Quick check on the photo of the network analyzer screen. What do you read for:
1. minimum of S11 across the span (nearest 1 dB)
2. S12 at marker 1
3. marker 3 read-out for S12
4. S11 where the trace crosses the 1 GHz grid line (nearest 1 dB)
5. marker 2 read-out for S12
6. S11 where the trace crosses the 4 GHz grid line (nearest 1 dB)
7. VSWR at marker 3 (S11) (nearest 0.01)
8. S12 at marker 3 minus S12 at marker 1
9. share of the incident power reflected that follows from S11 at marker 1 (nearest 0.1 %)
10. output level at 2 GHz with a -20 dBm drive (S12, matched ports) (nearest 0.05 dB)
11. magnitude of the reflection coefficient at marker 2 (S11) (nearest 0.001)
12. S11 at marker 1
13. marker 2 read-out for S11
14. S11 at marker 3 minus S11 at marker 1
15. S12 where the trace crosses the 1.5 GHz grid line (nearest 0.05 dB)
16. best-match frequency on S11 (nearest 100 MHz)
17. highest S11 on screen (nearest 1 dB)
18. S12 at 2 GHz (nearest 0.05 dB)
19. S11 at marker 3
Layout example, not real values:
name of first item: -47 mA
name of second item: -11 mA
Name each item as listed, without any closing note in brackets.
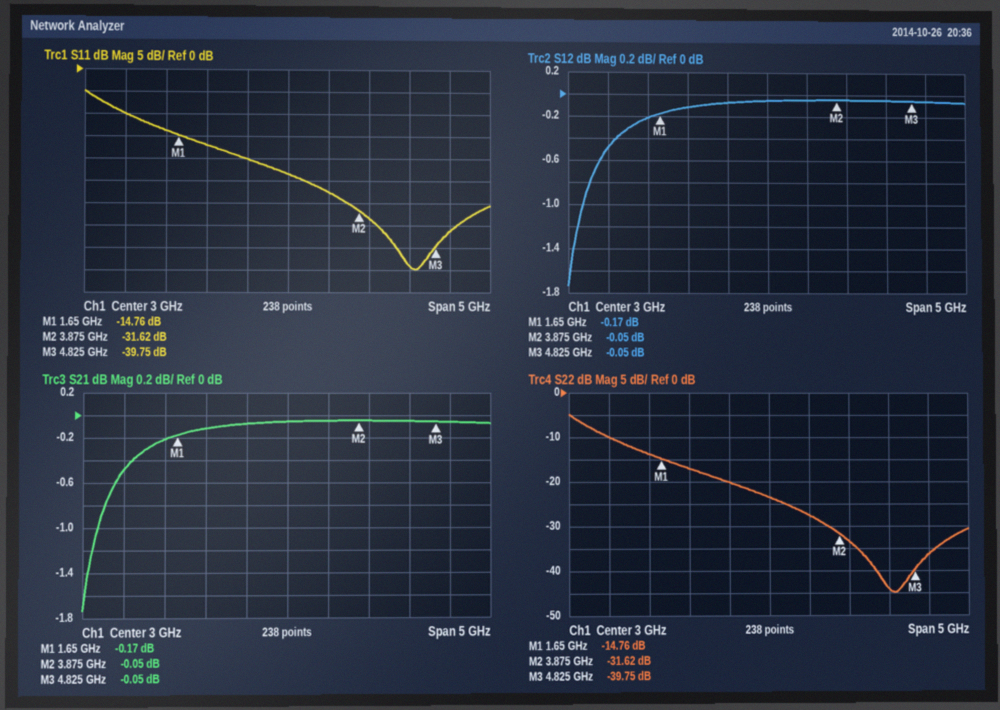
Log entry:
minimum of S11 across the span: -45 dB
S12 at marker 1: -0.17 dB
marker 3 read-out for S12: -0.05 dB
S11 where the trace crosses the 1 GHz grid line: -10 dB
marker 2 read-out for S12: -0.05 dB
S11 where the trace crosses the 4 GHz grid line: -33 dB
VSWR at marker 3 (S11): 1.02
S12 at marker 3 minus S12 at marker 1: 0.12 dB
share of the incident power reflected that follows from S11 at marker 1: 3.3 %
output level at 2 GHz with a -20 dBm drive (S12, matched ports): -20.10 dBm
magnitude of the reflection coefficient at marker 2 (S11): 0.026
S11 at marker 1: -14.76 dB
marker 2 read-out for S11: -31.62 dB
S11 at marker 3 minus S11 at marker 1: -24.99 dB
S12 where the trace crosses the 1.5 GHz grid line: -0.20 dB
best-match frequency on S11: 4.6 GHz
highest S11 on screen: -5 dB
S12 at 2 GHz: -0.10 dB
S11 at marker 3: -39.75 dB
